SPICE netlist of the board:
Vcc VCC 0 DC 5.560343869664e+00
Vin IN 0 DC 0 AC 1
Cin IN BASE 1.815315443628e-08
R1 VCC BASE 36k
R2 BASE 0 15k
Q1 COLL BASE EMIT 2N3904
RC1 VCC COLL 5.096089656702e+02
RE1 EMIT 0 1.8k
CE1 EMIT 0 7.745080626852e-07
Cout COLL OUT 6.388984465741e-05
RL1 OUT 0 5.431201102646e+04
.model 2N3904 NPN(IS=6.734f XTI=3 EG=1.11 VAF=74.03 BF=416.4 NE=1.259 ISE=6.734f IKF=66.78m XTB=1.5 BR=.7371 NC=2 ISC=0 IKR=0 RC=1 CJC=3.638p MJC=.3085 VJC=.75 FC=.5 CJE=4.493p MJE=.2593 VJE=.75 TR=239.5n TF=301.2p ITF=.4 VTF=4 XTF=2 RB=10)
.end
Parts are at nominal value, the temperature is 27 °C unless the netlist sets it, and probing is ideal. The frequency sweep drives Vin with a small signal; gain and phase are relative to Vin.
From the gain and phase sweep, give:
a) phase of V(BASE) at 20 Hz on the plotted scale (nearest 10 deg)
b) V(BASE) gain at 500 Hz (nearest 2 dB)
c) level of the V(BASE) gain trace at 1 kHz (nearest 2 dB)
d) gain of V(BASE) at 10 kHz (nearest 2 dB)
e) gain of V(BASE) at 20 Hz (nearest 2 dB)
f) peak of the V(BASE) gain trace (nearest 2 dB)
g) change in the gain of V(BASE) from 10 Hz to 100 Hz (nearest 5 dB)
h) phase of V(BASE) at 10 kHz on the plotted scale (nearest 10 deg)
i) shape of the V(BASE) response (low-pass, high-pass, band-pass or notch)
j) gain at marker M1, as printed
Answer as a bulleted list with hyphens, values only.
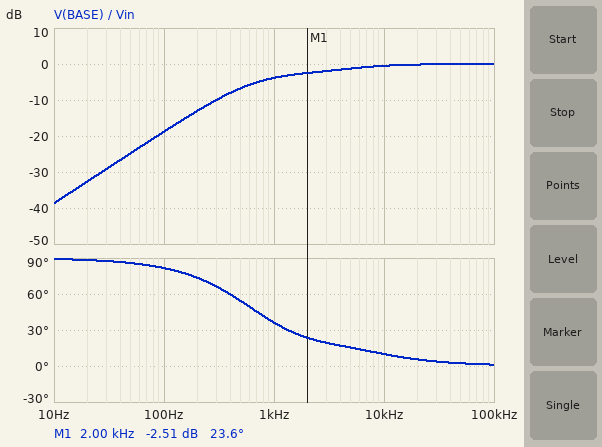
- 90 deg
- -6 dB
- -4 dB
- 0 dB
- -32 dB
- 0 dB
- 20 dB
- 10 deg
- high-pass
- -2.51 dB
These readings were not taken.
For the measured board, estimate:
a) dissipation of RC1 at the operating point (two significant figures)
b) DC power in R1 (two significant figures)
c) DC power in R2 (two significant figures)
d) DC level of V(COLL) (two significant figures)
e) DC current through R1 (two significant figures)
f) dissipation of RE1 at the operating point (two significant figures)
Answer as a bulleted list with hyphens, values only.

- 140 µW
- 440 µW
- 170 µW
- 5.3 V
- 110 µA
- 500 µW
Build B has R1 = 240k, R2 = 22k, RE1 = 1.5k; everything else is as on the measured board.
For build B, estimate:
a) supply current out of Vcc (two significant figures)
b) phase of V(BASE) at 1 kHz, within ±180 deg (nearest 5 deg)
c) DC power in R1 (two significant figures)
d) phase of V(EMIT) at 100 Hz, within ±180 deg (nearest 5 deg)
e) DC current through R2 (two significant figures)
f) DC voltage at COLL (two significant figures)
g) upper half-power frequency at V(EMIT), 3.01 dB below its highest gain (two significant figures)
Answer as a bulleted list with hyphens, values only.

- 22 µA
- 25 deg
- 110 µW
- 40 deg
- 21 µA
- 5.6 V
- 670 Hz
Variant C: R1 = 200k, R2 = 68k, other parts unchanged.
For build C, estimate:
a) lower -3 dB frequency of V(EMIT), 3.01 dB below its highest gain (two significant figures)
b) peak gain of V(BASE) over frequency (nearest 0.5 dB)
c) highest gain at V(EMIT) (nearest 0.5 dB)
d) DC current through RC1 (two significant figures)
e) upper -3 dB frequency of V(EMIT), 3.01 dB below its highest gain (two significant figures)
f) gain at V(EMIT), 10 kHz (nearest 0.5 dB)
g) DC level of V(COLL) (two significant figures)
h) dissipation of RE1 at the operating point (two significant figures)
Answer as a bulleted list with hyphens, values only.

- 150 Hz
- 0 dB
- -3.0 dB
- 350 µA
- 4.0 kHz
- -12.0 dB
- 5.4 V
- 220 µW
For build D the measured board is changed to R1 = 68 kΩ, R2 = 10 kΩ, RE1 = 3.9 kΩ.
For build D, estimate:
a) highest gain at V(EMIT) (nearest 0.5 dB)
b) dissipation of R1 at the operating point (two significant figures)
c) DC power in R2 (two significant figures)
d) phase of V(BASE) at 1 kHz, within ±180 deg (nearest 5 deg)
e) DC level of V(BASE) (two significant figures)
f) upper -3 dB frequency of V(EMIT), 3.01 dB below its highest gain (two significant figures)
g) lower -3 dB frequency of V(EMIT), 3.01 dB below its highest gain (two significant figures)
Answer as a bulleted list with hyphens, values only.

- -14.5 dB
- 350 µW
- 50 µW
- 45 deg
- 710 mV
- 1.6 kHz
- 200 Hz
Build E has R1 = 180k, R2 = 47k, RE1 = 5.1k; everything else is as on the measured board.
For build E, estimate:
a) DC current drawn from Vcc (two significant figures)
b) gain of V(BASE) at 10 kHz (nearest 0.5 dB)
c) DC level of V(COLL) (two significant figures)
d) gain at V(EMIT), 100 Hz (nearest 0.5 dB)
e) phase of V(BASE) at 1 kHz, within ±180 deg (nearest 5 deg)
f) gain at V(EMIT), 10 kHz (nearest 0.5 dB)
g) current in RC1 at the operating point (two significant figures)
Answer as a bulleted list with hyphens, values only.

- 120 µA
- 0 dB
- 5.5 V
- -9.5 dB
- 20 deg
- -22.0 dB
- 99 µA
